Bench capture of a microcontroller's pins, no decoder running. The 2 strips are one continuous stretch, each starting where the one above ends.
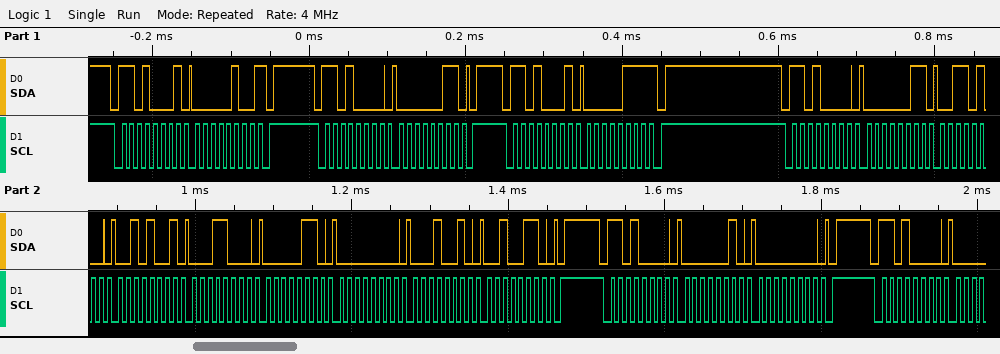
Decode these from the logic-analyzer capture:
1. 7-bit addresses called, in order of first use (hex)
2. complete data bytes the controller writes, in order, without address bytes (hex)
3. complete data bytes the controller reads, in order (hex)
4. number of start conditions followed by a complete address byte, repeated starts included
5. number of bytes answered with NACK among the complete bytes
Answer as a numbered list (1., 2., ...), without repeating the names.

1. 0x68
2. 03 03 34 29 18 06 00 12 26 02 00
3. 04 07
4. 6
5. 2
